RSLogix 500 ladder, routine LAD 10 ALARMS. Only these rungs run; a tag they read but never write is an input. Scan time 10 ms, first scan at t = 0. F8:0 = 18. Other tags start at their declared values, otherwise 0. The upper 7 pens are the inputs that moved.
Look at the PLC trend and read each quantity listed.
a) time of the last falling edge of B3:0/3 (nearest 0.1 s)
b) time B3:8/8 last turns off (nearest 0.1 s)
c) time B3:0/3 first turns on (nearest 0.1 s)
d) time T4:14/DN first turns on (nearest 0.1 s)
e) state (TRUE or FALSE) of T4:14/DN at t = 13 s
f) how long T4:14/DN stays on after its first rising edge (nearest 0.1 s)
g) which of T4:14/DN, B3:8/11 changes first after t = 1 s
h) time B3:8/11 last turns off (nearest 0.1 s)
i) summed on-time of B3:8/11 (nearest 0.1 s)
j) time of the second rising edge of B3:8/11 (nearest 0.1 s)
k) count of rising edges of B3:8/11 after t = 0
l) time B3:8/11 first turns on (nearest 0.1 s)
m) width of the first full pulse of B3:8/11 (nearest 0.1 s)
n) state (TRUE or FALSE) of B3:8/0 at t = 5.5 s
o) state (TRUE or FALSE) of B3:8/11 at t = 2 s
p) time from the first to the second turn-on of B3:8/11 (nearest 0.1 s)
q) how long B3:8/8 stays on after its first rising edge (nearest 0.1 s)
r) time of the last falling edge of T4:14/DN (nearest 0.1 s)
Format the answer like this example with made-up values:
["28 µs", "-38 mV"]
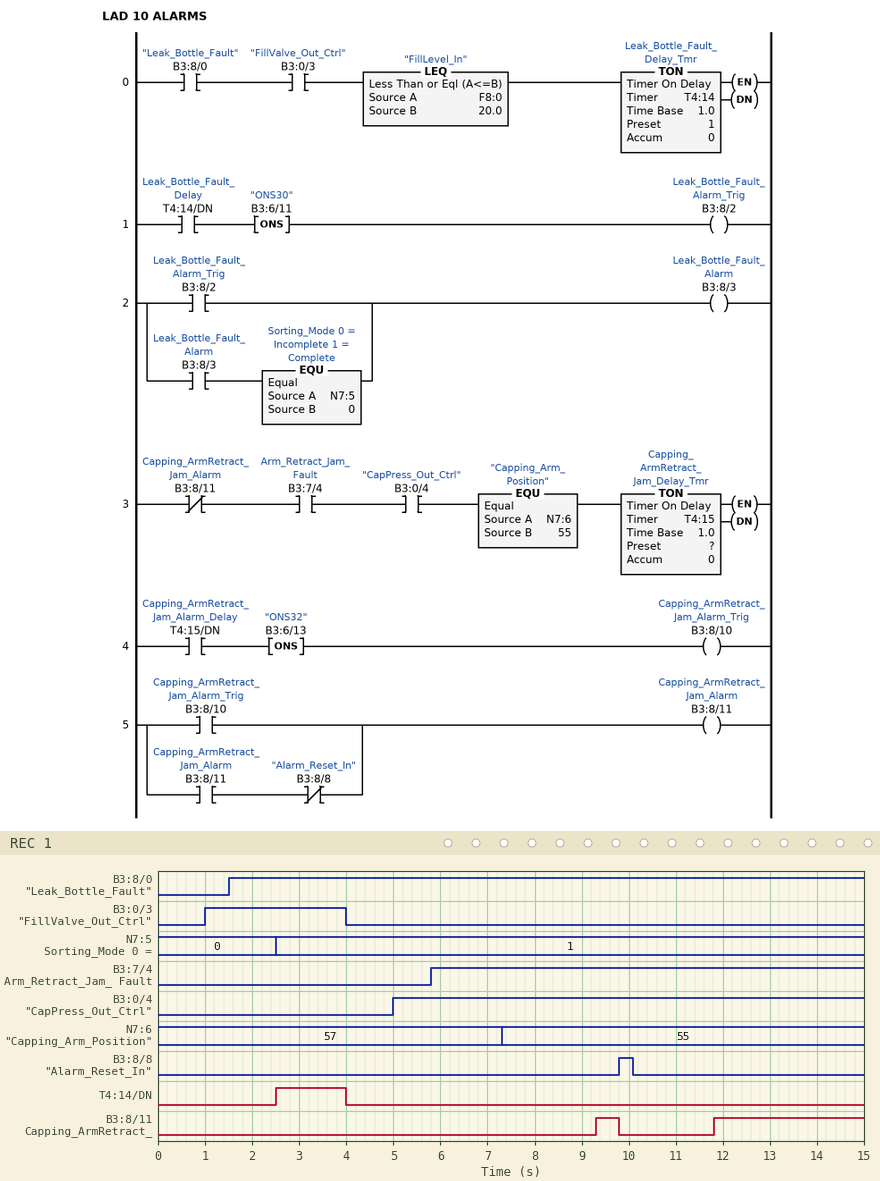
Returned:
["4.0 s", "10.1 s", "1.0 s", "2.5 s", "FALSE", "1.5 s", "T4:14/DN", "9.8 s", "3.7 s", "11.8 s", "2", "9.3 s", "0.5 s", "TRUE", "FALSE", "2.5 s", "0.3 s", "4.0 s"]
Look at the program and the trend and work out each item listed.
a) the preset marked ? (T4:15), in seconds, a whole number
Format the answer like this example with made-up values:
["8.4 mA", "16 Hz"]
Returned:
["2 s"]
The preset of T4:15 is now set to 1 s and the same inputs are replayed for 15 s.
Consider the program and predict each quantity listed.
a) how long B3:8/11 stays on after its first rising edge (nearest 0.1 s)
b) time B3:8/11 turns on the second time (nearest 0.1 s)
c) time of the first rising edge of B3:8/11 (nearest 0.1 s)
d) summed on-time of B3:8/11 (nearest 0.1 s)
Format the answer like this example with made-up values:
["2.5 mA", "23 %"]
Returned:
["1.5 s", "10.8 s", "8.3 s", "5.7 s"]
